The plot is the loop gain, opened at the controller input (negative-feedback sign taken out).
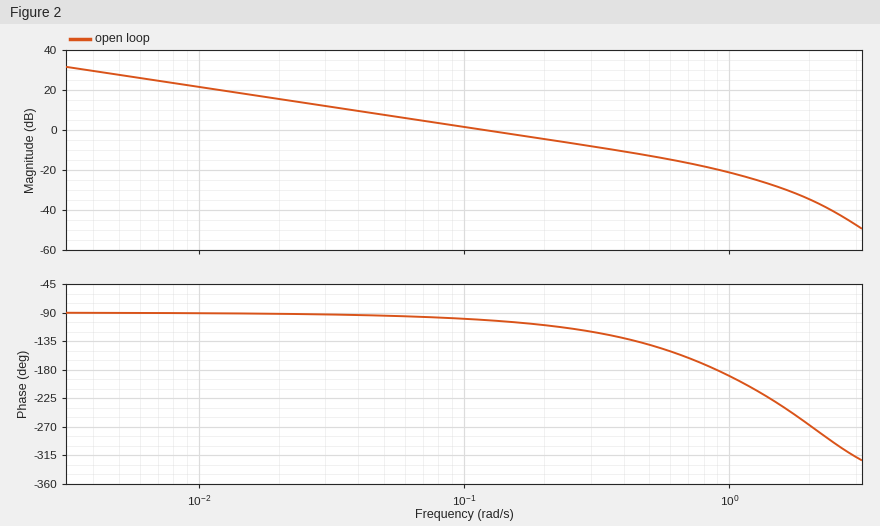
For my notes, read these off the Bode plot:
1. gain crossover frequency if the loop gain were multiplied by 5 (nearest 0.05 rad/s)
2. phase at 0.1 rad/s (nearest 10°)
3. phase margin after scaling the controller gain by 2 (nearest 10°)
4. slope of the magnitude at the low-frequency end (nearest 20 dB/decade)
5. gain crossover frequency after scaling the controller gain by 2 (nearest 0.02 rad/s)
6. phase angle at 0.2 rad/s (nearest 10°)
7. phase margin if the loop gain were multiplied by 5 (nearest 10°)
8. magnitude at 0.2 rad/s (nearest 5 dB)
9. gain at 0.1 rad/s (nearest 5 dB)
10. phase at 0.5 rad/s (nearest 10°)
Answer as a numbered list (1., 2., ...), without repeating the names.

1. 0.55 rad/s
2. -100°
3. 70°
4. -20 dB/decade
5. 0.24 rad/s
6. -110°
7. 30°
8. -5 dB
9. 0 dB
10. -140°
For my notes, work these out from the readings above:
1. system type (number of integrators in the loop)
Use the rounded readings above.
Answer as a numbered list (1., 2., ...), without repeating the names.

1. 1
